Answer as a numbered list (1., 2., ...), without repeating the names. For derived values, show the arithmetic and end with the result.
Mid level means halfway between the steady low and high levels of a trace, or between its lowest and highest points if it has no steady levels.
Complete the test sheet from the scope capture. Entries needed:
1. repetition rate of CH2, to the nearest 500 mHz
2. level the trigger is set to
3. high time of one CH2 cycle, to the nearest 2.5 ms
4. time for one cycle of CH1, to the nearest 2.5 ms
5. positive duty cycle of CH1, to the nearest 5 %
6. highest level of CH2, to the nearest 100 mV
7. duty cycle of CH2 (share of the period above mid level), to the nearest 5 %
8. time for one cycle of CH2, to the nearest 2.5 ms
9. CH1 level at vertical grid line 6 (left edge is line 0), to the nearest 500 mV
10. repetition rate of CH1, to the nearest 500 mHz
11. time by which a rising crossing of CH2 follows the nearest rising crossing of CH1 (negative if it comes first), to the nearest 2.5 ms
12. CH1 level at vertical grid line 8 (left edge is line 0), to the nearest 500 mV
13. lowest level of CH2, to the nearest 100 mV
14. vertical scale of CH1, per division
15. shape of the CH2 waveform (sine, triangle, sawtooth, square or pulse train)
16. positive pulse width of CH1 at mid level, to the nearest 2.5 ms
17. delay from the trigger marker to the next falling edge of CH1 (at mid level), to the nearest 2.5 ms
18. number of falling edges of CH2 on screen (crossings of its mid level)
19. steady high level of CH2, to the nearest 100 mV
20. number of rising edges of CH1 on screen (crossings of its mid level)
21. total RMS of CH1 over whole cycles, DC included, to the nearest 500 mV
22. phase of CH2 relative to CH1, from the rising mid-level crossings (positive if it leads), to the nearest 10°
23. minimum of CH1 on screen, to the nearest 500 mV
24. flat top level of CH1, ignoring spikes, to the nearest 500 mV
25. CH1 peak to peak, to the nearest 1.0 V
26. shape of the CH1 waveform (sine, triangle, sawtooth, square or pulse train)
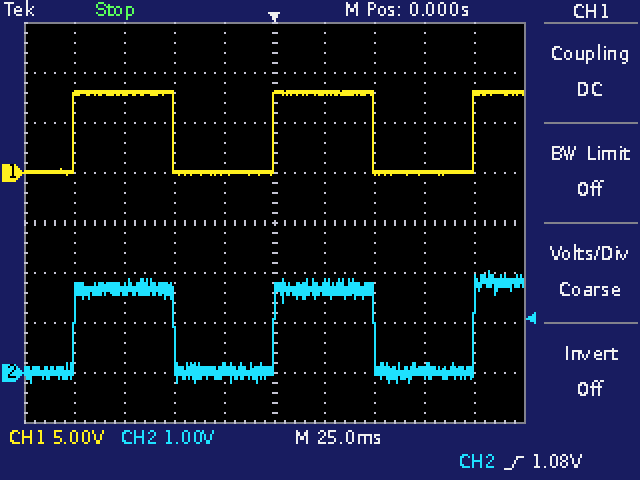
1. 1 / 100.0 ms ≈ 10.0 Hz
2. 1.08 V
3. 50.0 ms
4. 100.0 ms
5. 50.0 ms / 100.0 ms ≈ 50 %
6. 2.0 V
7. 50.0 ms / 100.0 ms ≈ 50 %
8. 100.0 ms
9. 8.0 V
10. 1 / 100.0 ms ≈ 10.0 Hz
11. 0.0 ms
12. 0.0 V
13. -200 mV
14. 5 V
15. square
16. 50.0 ms
17. 50.0 ms
18. 2
19. 1.7 V
20. 3
21. √(0.5 × (8.0 V)² + 0.5 × (0.0 V)²) ≈ 5.66 V, so 5.5 V to the nearest 500 mV
22. −360° × (0.0 ms) / 100.0 ms ≈ 0°
23. 0.0 V
24. 8.0 V
25. 8.0 V
26. square
